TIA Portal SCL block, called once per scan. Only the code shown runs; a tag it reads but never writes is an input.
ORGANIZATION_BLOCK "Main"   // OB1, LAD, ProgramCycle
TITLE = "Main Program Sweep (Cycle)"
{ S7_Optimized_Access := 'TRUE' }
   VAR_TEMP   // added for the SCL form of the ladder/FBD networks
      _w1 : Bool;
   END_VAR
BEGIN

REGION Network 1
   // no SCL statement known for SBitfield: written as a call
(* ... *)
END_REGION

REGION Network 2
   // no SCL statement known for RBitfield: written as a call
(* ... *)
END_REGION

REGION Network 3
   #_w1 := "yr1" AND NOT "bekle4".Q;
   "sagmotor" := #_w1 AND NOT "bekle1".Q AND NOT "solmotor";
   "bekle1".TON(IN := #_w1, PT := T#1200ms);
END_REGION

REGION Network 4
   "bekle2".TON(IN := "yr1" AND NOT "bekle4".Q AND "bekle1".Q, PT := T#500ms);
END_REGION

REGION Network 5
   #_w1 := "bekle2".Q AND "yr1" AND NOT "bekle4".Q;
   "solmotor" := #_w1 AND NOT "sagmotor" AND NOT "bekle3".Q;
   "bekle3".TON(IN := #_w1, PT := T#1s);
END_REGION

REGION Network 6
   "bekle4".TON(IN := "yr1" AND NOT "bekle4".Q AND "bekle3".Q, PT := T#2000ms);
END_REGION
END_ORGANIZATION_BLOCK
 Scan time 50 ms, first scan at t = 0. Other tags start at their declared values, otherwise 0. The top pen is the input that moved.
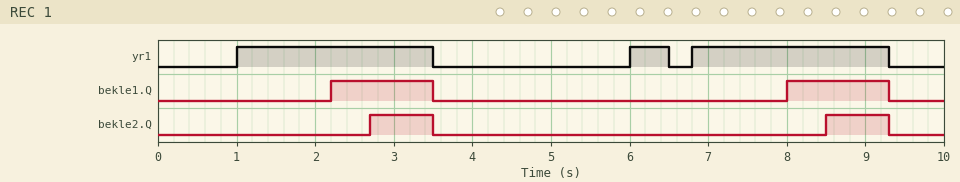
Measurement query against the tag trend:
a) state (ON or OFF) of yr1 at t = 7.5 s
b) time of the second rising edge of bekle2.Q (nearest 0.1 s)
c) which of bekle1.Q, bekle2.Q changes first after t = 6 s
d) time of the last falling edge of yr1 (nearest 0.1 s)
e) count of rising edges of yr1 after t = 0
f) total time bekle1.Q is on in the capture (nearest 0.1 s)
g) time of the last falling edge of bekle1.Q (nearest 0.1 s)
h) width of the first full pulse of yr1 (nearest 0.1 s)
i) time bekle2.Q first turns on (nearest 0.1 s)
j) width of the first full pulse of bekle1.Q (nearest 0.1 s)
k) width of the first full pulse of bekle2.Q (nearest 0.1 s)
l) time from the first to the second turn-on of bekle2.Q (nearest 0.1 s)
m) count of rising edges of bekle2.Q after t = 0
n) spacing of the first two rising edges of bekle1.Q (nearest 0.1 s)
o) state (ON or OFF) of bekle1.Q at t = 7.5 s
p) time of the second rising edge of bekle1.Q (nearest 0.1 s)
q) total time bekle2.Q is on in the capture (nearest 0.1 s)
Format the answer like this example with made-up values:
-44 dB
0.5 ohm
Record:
ON
8.5 s
bekle1.Q
9.3 s
3
2.6 s
9.3 s
2.5 s
2.7 s
1.3 s
0.8 s
5.8 s
2
5.8 s
OFF
8.0 s
1.6 s
